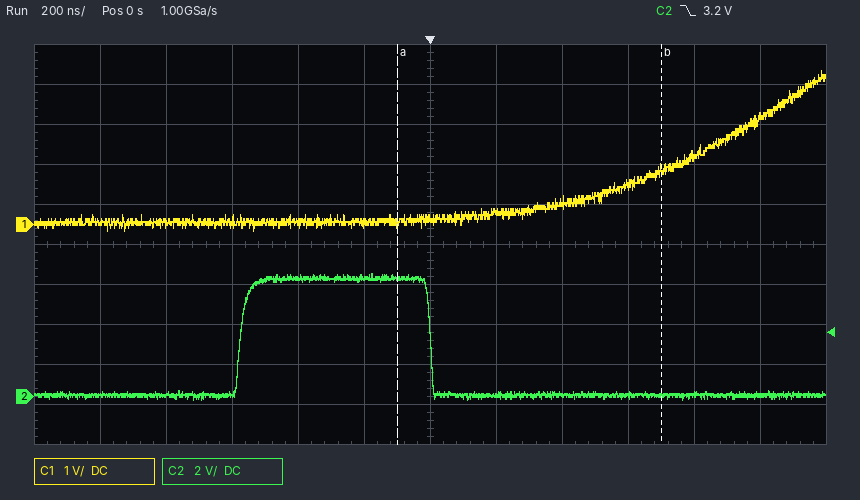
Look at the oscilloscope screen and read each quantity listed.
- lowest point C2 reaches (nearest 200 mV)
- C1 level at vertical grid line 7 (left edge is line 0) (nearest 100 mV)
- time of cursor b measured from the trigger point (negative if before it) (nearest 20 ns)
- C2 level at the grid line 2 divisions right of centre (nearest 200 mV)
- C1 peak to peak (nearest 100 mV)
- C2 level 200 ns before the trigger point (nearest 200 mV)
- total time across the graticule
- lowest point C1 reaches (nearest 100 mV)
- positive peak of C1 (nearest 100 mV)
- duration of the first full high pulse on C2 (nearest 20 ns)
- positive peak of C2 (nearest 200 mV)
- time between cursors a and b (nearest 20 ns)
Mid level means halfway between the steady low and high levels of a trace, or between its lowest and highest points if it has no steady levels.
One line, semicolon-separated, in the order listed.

-200 mV; 300 mV; +700 ns; 200 mV; 4.0 V; 6.0 V; 2.4 µs; -200 mV; 3.8 V; 580 ns; 6.2 V; 800 ns
